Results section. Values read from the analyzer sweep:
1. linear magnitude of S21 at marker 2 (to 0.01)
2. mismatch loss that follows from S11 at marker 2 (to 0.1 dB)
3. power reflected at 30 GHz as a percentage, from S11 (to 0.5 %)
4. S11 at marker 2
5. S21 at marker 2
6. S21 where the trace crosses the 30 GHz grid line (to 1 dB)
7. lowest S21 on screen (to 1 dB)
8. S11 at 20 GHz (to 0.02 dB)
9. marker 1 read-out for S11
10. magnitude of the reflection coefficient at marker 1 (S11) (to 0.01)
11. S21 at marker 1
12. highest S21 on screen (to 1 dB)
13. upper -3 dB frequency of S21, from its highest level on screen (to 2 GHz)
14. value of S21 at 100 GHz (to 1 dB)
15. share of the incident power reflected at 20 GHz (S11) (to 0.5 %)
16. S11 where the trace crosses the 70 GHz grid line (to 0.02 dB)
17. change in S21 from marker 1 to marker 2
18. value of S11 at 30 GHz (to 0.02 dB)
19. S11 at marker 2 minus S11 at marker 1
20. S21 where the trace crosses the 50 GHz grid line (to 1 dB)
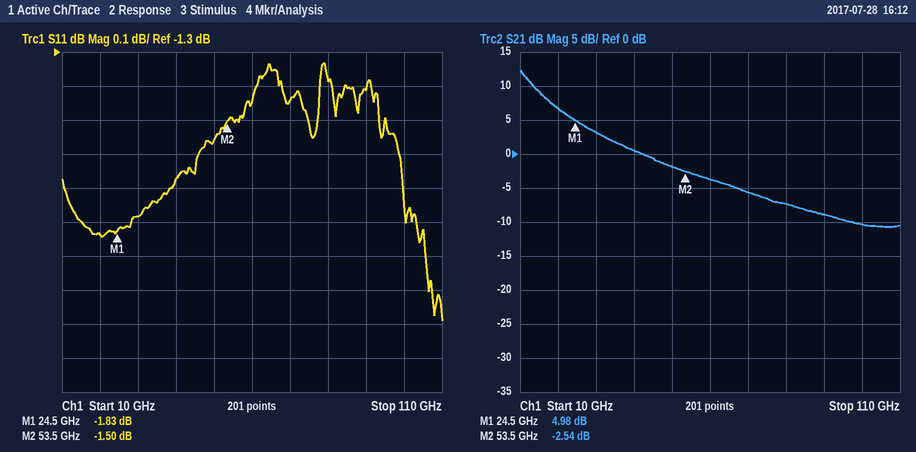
0.75
5.3 dB
66.5 %
-1.50 dB
-2.54 dB
3 dB
-11 dB
-1.84 dB
-1.83 dB
0.81
4.98 dB
12 dB
14 GHz
-10 dB
65.5 %
-1.44 dB
-7.52 dB
-1.78 dB
0.33 dB
-2 dB
